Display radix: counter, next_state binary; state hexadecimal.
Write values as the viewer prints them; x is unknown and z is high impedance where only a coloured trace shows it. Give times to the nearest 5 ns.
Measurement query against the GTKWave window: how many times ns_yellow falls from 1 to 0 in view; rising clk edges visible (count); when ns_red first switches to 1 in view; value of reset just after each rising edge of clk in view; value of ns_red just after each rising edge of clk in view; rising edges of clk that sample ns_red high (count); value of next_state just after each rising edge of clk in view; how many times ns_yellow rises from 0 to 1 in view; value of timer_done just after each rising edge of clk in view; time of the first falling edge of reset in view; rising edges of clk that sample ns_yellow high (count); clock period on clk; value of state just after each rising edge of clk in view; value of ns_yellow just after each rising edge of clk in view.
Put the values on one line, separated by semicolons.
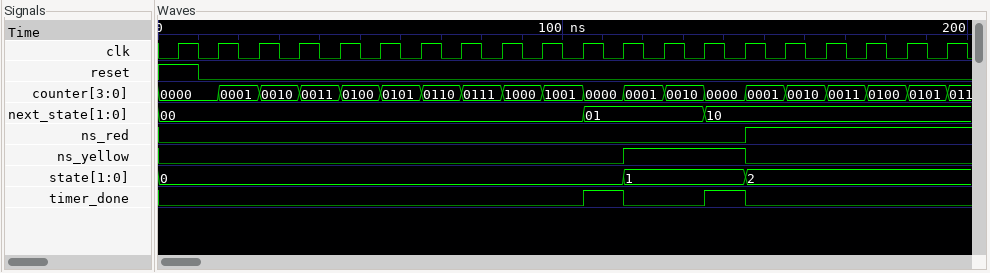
1; 20; 145 ns; 1 0 0 0 0 0 0 0 0 0 0 0 0 0 0 0 0 0 0 0; 0 0 0 0 0 0 0 0 0 0 0 0 0 0 1 1 1 1 1 1; 5; 00, 00, 00, 00, 00, 00, 00, 00, 00, 00, 01, 01, 01, 10, 10, 10, 10, 10, 10, 10; 1; 0 0 0 0 0 0 0 0 0 0 1 0 0 1 0 0 0 0 0 0; 10 ns; 3; 10 ns; 0, 0, 0, 0, 0, 0, 0, 0, 0, 0, 0, 1, 1, 1, 2, 2, 2, 2, 2, 2; 0 0 0 0 0 0 0 0 0 0 0 1 1 1 0 0 0 0 0 0
